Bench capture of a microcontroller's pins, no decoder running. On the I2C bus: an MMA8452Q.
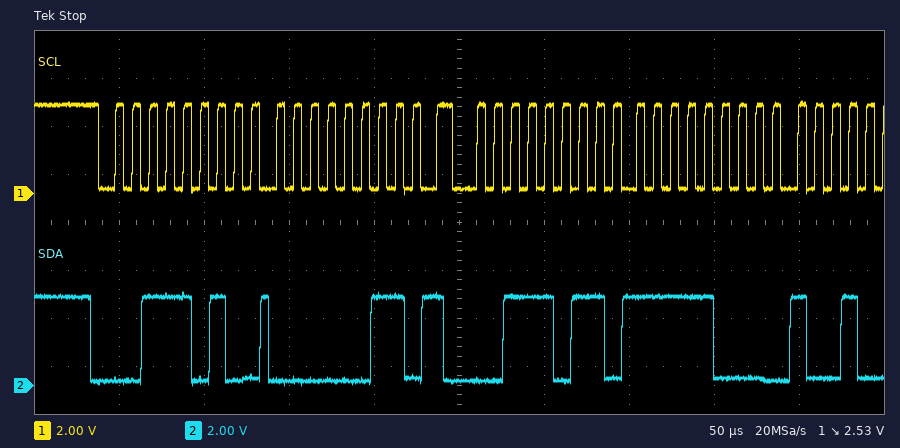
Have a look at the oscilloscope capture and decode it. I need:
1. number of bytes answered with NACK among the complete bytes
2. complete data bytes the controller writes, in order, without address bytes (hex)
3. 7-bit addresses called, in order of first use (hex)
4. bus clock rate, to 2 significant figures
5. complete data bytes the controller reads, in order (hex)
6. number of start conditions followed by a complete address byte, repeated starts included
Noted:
0
03
0x1D
100 kHz
F8
2
